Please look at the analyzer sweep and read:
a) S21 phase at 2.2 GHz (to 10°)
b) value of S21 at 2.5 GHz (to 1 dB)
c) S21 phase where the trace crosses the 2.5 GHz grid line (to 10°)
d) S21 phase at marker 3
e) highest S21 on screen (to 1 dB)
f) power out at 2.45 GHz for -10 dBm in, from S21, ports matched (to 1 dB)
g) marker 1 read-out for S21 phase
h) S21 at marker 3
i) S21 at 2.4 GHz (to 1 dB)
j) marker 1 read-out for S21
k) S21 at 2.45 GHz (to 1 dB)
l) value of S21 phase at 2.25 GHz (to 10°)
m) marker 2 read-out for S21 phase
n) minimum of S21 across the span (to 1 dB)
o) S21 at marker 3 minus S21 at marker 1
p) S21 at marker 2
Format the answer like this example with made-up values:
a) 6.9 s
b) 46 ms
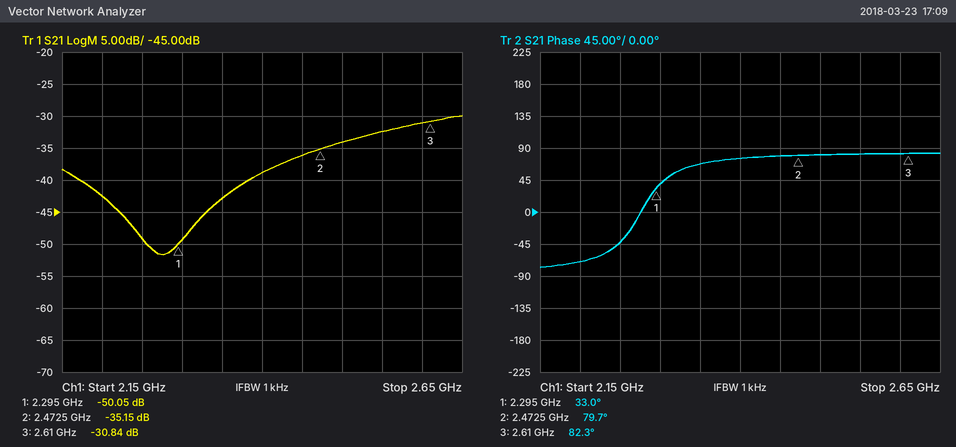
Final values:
a) -70°
b) -34 dB
c) 80°
d) 82.3°
e) -30 dB
f) -46 dBm
g) 33.0°
h) -30.84 dB
i) -39 dB
j) -50.05 dB
k) -36 dB
l) -40°
m) 79.7°
n) -52 dB
o) 19.21 dB
p) -35.15 dB
